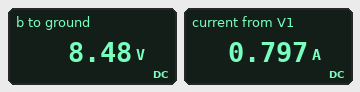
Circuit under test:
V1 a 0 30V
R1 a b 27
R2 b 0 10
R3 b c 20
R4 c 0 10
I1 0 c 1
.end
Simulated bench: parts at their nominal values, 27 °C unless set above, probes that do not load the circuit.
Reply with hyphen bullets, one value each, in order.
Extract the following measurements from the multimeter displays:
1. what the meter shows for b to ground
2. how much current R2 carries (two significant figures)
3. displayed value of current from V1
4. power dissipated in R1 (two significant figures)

- 8.48 V
- 850 mA
- 0.797 A
- 17 W
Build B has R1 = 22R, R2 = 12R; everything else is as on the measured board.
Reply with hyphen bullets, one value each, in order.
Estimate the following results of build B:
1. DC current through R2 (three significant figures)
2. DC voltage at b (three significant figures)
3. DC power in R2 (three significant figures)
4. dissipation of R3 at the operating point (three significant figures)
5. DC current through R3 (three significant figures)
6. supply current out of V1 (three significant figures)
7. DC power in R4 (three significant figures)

- 872 mA
- 10.5 V
- 9.13 W
- 4.85 mW
- 15.6 mA
- 888 mA
- 10.3 W
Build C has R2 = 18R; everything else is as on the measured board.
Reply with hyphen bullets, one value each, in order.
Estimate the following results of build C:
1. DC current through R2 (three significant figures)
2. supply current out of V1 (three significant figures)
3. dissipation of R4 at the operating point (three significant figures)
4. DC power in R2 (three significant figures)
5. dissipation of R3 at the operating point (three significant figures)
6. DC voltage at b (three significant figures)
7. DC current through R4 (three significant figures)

- 637 mA
- 686 mA
- 11.0 W
- 7.31 W
- 48.1 mW
- 11.5 V
- 1.05 A
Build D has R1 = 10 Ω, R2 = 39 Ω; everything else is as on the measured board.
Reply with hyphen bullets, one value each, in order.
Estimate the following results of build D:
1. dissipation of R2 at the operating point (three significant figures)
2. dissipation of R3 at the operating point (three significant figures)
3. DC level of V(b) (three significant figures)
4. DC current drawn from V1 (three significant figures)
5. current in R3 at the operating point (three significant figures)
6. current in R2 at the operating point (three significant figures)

- 11.3 W
- 2.67 W
- 21.0 V
- 903 mA
- 366 mA
- 538 mA
